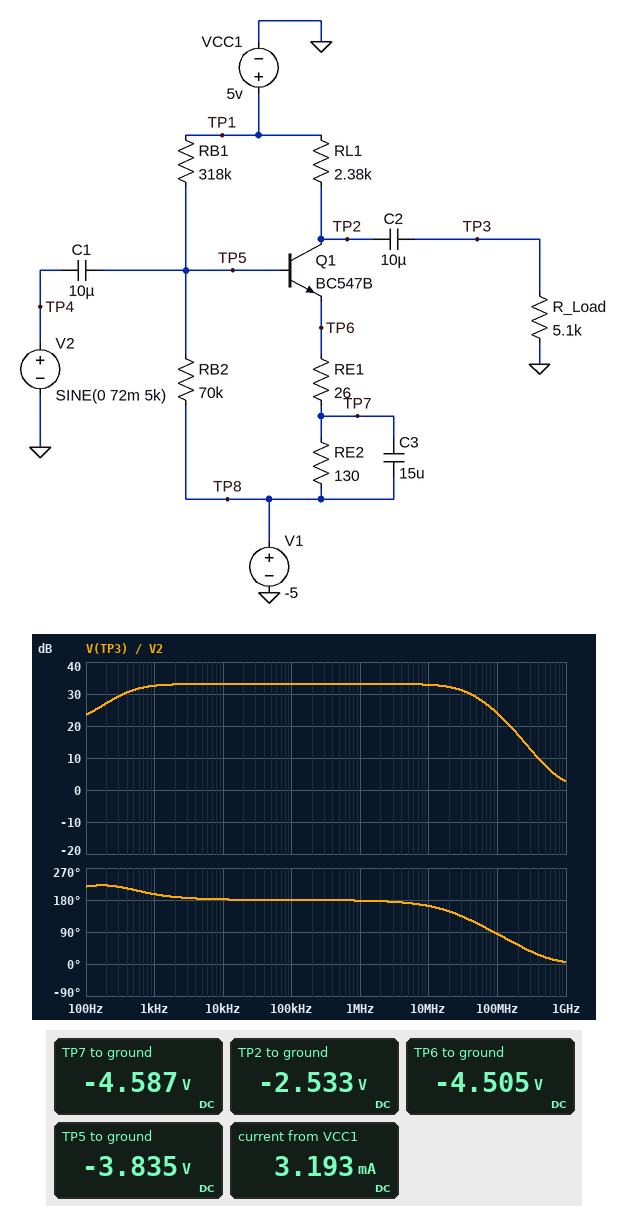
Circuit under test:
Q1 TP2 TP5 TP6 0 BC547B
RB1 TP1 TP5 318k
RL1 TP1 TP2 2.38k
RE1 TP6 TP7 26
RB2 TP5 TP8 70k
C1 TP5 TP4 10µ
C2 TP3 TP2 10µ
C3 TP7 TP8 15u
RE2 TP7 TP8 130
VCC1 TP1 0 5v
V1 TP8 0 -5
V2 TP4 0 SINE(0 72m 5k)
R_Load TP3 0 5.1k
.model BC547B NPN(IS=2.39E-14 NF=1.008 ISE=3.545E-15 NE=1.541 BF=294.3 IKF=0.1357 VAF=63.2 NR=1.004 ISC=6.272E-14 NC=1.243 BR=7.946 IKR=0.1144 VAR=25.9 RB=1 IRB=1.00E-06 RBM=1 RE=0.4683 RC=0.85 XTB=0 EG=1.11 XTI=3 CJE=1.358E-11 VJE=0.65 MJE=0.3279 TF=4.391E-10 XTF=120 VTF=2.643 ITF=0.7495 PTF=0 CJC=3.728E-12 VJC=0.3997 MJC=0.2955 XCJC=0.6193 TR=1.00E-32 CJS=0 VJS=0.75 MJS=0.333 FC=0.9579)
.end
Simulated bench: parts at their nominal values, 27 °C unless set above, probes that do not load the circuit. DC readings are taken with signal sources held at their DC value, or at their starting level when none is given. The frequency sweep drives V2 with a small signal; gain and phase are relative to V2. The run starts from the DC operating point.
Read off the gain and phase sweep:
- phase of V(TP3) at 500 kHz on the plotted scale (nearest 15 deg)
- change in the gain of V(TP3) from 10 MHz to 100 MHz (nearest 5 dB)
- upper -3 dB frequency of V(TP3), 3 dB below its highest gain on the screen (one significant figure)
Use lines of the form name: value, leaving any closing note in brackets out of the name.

phase of V(TP3) at 500 kHz on the plotted scale: 180 deg
change in the gain of V(TP3) from 10 MHz to 100 MHz: -10 dB
upper -3 dB frequency of V(TP3), 3 dB below its highest gain on the screen: 40 MHz
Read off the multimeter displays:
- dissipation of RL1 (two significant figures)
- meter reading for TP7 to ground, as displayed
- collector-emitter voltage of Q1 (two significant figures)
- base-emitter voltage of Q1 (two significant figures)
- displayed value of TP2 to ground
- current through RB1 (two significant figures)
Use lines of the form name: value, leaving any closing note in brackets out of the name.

dissipation of RL1: 24 mW
meter reading for TP7 to ground, as displayed: -4.587 V
collector-emitter voltage of Q1: 2.0 V
base-emitter voltage of Q1: 670 mV
displayed value of TP2 to ground: -2.533 V
current through RB1: 28 µA
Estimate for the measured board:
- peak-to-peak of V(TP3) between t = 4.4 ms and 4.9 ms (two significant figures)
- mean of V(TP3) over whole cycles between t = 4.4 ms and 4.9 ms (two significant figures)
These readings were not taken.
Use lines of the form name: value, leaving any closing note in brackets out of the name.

peak-to-peak of V(TP3) between t = 4.4 ms and 4.9 ms: 5.2 V
mean of V(TP3) over whole cycles between t = 4.4 ms and 4.9 ms: 450 mV
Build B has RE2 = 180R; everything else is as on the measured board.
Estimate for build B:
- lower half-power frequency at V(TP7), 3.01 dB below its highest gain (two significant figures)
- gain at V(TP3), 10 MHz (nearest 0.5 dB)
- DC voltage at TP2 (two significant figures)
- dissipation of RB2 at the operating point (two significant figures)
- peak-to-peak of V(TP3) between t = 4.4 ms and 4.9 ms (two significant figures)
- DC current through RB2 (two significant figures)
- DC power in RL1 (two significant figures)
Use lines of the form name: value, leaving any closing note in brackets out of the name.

lower half-power frequency at V(TP7), 3.01 dB below its highest gain: 560 mHz
gain at V(TP3), 10 MHz: 32.5 dB
DC voltage at TP2: -1.7 V
dissipation of RB2 at the operating point: 22 µW
peak-to-peak of V(TP3) between t = 4.4 ms and 4.9 ms: 5.6 V
DC current through RB2: 18 µA
DC power in RL1: 19 mW
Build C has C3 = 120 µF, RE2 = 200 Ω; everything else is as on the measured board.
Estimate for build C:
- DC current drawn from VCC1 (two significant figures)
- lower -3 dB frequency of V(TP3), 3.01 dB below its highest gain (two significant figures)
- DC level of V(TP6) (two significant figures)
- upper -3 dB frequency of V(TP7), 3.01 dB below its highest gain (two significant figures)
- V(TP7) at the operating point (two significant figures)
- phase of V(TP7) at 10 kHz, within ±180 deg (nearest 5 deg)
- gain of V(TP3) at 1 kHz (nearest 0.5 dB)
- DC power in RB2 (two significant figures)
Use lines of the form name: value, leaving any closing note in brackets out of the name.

DC current drawn from VCC1: 2.7 mA
lower -3 dB frequency of V(TP3), 3.01 dB below its highest gain: 43 Hz
DC level of V(TP6): -4.4 V
upper -3 dB frequency of V(TP7), 3.01 dB below its highest gain: 45 Hz
V(TP7) at the operating point: -4.5 V
phase of V(TP7) at 10 kHz, within ±180 deg: -90 deg
gain of V(TP3) at 1 kHz: 33.0 dB
DC power in RB2: 23 µW
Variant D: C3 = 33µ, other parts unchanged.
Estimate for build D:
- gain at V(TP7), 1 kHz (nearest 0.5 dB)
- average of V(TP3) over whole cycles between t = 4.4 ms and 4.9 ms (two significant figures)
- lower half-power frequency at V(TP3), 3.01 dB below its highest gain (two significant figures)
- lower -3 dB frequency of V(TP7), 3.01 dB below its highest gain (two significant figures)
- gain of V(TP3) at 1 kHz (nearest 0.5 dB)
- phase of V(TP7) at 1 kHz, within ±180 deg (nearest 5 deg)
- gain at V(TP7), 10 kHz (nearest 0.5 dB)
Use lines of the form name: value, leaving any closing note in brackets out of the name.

gain at V(TP7), 1 kHz: -17.5 dB
average of V(TP3) over whole cycles between t = 4.4 ms and 4.9 ms: 490 mV
lower half-power frequency at V(TP3), 3.01 dB below its highest gain: 170 Hz
lower -3 dB frequency of V(TP7), 3.01 dB below its highest gain: 650 mHz
gain of V(TP3) at 1 kHz: 33.0 dB
phase of V(TP7) at 1 kHz, within ±180 deg: -80 deg
gain at V(TP7), 10 kHz: -37.5 dB
